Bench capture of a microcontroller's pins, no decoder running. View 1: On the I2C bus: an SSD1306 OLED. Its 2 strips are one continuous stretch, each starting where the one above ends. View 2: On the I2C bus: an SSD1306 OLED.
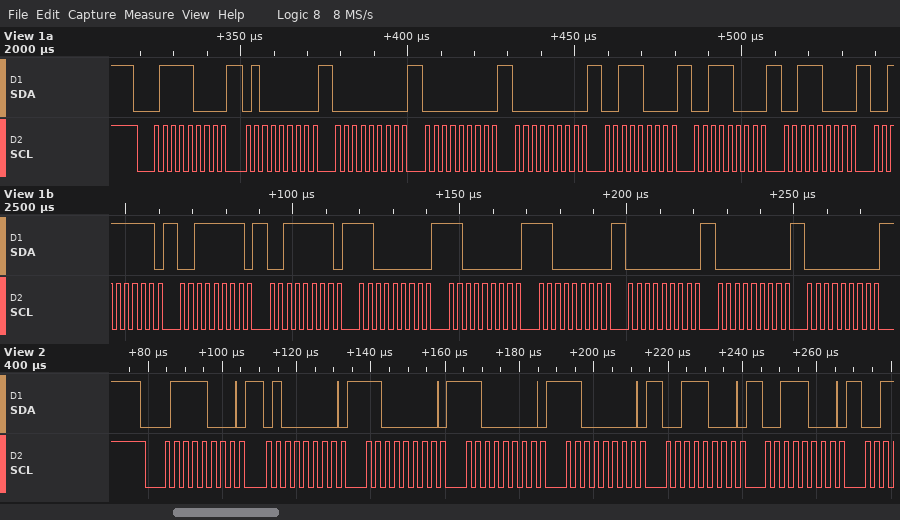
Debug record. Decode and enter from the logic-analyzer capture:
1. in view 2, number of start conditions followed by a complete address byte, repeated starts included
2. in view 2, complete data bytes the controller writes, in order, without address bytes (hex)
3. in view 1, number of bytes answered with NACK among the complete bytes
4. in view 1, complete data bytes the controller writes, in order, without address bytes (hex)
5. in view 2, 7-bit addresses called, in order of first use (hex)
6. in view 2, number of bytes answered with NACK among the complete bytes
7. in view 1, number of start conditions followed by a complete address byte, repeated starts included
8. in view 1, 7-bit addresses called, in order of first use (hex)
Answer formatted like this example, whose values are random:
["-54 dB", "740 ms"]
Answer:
["1", "40 C0 C0 C0 38 38", "0", "40 00 00 00 38 38 38 3F 3F 3F C0 C0 C0 00 00 00", "0x3C", "0", "1", "0x3C"]
